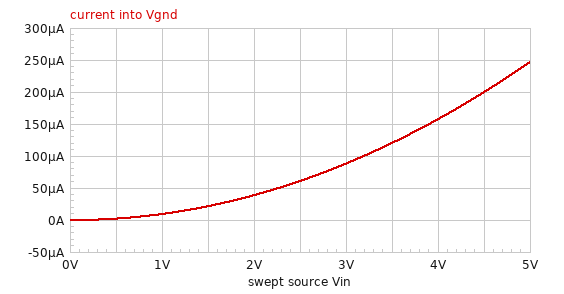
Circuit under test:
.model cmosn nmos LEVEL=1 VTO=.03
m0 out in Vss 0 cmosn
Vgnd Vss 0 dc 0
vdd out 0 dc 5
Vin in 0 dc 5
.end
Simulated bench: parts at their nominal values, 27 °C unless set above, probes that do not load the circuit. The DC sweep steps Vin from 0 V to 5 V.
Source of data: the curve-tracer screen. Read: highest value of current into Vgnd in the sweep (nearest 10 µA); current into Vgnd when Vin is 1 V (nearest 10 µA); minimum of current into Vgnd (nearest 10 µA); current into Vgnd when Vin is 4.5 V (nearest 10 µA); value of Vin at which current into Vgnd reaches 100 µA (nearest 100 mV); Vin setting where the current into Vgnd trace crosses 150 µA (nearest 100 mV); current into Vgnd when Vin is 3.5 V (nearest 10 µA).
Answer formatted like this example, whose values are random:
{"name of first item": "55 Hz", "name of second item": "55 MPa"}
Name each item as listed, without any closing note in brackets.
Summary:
{"highest value of current into Vgnd in the sweep": "250 µA", "current into Vgnd when Vin is 1 V": "10 µA", "minimum of current into Vgnd": "0 A", "current into Vgnd when Vin is 4.5 V": "200 µA", "value of Vin at which current into Vgnd reaches 100 µA": "3.2 V", "Vin setting where the current into Vgnd trace crosses 150 µA": "3.9 V", "current into Vgnd when Vin is 3.5 V": "120 µA"}
